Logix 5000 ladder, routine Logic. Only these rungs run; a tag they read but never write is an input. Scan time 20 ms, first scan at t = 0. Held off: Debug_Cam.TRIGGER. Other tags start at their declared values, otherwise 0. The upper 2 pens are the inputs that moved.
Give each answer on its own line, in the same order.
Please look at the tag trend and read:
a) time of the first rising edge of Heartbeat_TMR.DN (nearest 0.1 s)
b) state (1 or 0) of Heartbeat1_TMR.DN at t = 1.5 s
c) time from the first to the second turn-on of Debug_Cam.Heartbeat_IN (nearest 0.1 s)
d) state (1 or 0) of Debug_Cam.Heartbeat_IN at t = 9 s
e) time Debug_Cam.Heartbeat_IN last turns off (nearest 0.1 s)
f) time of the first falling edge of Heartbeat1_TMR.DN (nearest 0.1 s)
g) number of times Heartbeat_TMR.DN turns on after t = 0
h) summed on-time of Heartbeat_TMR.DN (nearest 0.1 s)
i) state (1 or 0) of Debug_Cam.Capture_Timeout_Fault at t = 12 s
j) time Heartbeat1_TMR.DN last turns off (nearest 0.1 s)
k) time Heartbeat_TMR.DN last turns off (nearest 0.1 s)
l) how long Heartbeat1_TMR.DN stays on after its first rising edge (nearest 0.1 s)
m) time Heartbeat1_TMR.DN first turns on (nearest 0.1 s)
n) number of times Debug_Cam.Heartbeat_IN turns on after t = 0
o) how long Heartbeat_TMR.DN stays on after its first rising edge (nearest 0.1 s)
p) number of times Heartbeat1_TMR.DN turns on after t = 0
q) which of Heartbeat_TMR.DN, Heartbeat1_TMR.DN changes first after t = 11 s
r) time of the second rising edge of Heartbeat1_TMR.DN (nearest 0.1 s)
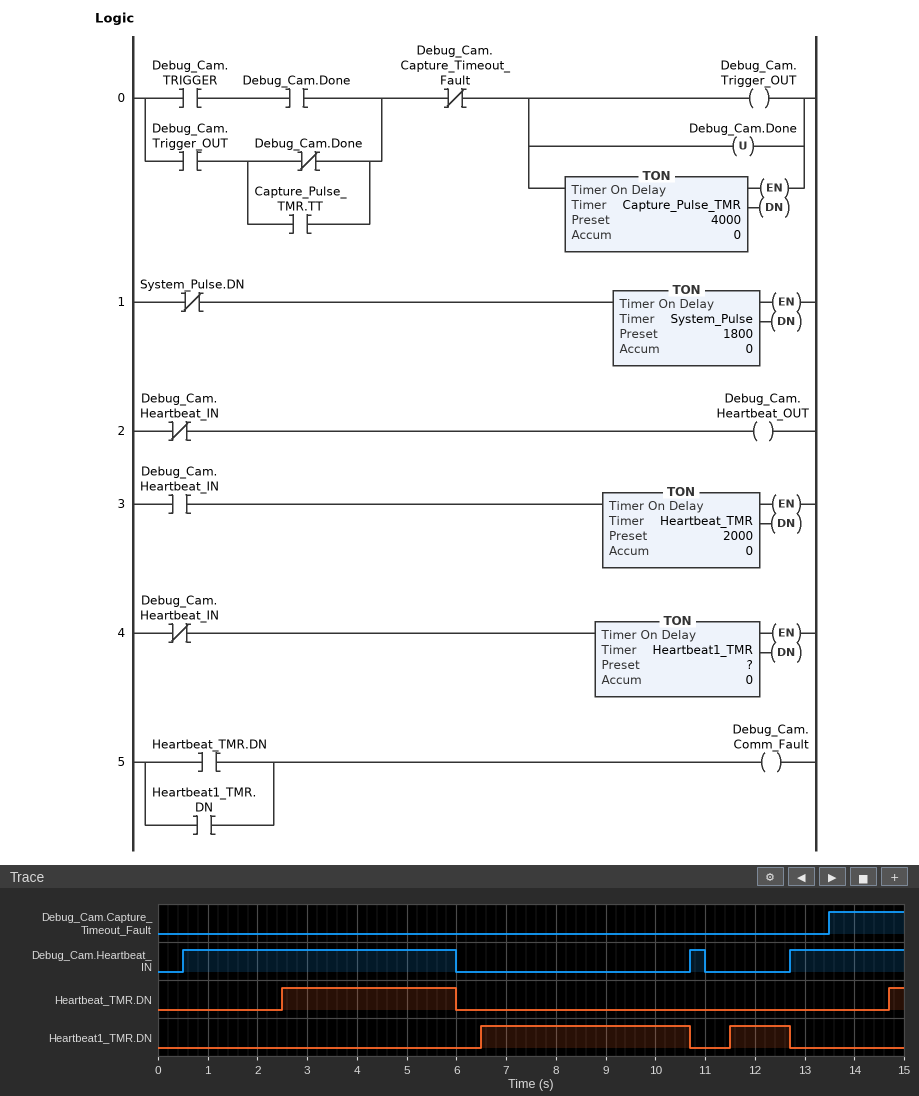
2.5 s
0
10.2 s
0
11.0 s
10.7 s
2
3.8 s
0
12.7 s
6.0 s
4.2 s
6.5 s
3
3.5 s
2
Heartbeat1_TMR.DN
11.5 s
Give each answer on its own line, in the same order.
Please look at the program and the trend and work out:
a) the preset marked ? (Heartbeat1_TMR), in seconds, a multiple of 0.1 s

0.5 s
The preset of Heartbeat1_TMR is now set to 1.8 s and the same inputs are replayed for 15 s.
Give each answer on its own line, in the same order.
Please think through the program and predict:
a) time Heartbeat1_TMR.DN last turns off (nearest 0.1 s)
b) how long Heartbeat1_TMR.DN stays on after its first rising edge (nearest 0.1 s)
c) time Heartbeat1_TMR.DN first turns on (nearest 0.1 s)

10.7 s
2.9 s
7.8 s
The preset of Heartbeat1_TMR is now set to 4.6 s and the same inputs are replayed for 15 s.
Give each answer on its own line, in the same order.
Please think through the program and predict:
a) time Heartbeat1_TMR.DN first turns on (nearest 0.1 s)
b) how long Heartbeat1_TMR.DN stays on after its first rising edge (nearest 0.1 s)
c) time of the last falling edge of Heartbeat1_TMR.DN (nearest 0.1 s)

10.6 s
0.1 s
10.7 s
